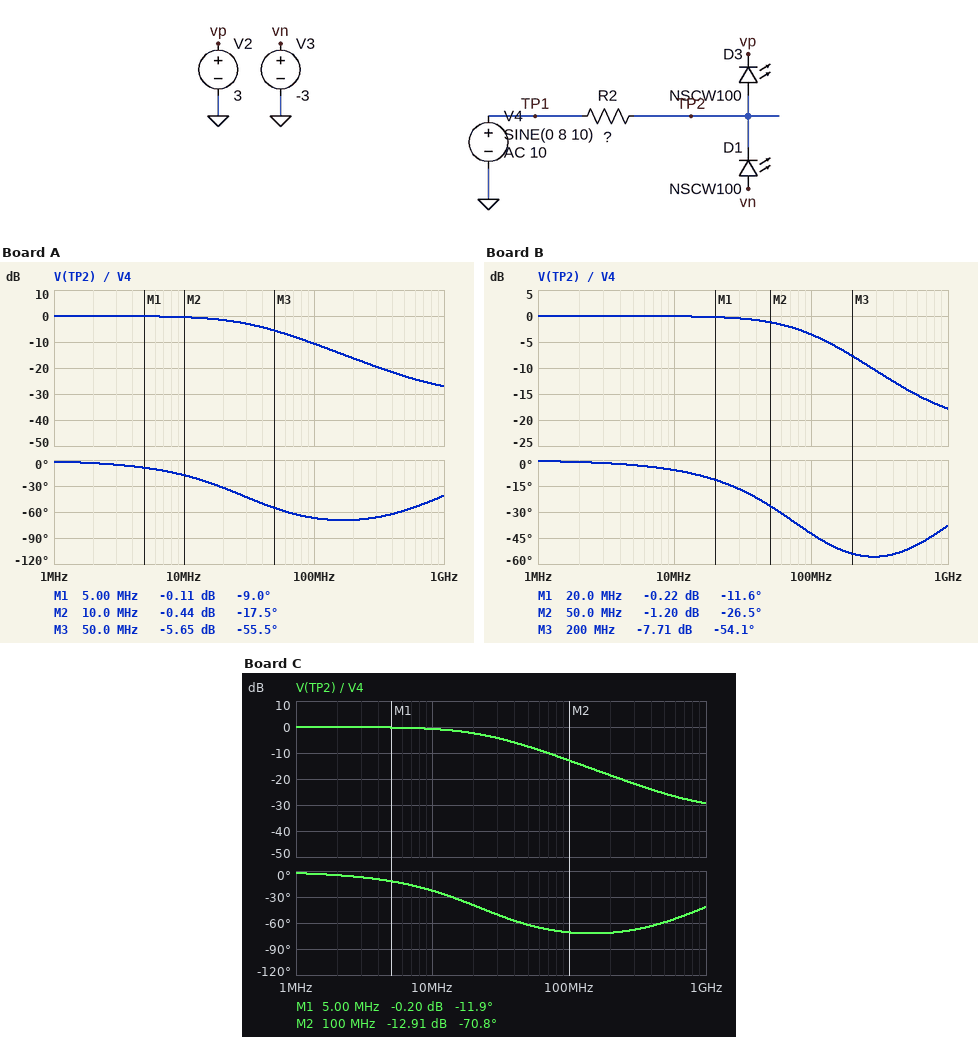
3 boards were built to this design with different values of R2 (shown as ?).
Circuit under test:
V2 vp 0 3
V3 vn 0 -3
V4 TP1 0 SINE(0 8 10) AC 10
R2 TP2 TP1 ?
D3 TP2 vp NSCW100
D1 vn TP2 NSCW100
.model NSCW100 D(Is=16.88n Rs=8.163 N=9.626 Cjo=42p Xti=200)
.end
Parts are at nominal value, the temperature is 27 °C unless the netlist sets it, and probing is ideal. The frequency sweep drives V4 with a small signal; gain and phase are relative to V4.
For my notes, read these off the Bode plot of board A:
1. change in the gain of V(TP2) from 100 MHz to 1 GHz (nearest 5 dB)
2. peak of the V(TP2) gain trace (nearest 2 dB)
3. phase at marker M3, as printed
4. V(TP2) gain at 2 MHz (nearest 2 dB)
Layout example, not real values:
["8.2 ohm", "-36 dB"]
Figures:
["-15 dB", "0 dB", "-55.5 deg", "0 dB"]
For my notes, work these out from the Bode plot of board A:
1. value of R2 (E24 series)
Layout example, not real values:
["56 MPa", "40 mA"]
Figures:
["120 Ω"]
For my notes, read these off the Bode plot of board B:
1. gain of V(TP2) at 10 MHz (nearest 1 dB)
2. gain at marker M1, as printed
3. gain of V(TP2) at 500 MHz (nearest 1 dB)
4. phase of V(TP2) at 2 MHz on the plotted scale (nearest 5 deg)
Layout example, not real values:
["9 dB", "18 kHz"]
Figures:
["0 dB", "-0.22 dB", "-14 dB", "0 deg"]
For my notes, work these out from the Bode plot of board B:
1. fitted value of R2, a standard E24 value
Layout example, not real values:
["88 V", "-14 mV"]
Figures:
["39 Ω"]
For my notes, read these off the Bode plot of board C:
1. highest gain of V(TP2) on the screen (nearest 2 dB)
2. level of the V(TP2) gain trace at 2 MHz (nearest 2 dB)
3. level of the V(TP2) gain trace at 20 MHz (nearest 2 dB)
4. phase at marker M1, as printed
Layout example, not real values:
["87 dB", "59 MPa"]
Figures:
["0 dB", "0 dB", "-2 dB", "-11.9 deg"]
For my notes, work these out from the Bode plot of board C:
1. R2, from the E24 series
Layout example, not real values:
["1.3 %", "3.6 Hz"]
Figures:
["160 Ω"]
